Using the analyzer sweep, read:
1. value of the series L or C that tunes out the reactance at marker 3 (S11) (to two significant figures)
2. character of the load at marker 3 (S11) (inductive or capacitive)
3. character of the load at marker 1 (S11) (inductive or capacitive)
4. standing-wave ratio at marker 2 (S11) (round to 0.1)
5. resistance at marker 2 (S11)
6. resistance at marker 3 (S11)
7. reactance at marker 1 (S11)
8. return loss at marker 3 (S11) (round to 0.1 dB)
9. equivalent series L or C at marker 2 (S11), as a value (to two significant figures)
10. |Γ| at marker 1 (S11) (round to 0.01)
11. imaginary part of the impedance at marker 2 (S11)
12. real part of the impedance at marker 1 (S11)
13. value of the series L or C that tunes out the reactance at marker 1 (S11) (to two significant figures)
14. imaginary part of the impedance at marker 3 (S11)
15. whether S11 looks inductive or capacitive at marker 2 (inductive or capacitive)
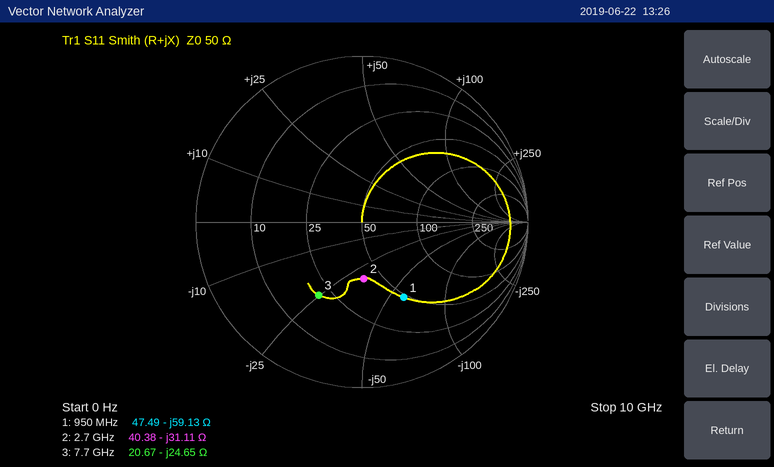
510 pH
capacitive
capacitive
2.0
40.38 Ω
20.67 Ω
-59.13 Ω
5.8 dB
1.9 pF
0.52
-31.11 Ω
47.49 Ω
9.9 nH
-24.65 Ω
capacitive
